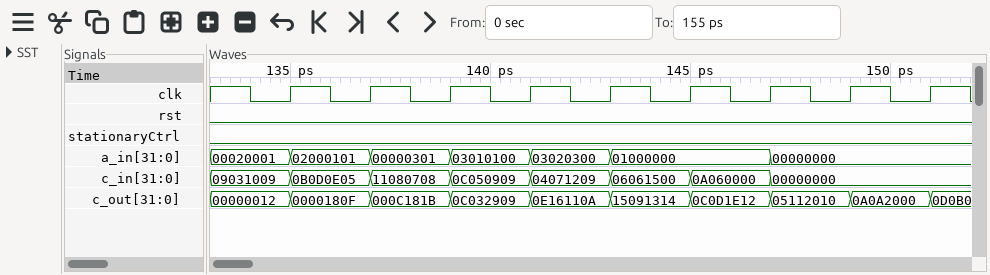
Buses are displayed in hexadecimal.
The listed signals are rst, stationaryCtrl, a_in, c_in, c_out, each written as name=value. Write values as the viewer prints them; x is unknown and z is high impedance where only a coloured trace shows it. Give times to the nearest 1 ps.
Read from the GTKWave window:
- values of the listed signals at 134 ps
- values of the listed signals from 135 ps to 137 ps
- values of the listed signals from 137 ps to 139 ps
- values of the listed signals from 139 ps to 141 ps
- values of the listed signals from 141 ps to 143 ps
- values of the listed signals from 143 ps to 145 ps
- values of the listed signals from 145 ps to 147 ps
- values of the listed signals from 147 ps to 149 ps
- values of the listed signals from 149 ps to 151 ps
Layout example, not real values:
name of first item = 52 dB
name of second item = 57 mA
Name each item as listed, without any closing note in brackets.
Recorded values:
values of the listed signals at 134 ps = rst=0, stationaryCtrl=0, a_in=00020001, c_in=09031009, c_out=00000012
values of the listed signals from 135 ps to 137 ps = rst=0, stationaryCtrl=0, a_in=02000101, c_in=0B0D0E05, c_out=0000180F
values of the listed signals from 137 ps to 139 ps = rst=0, stationaryCtrl=0, a_in=00000301, c_in=11080708, c_out=000C181B
values of the listed signals from 139 ps to 141 ps = rst=0, stationaryCtrl=0, a_in=03010100, c_in=0C050909, c_out=0C032909
values of the listed signals from 141 ps to 143 ps = rst=0, stationaryCtrl=0, a_in=03020300, c_in=04071209, c_out=0E16110A
values of the listed signals from 143 ps to 145 ps = rst=0, stationaryCtrl=0, a_in=01000000, c_in=06061500, c_out=15091314
values of the listed signals from 145 ps to 147 ps = rst=0, stationaryCtrl=0, a_in=01000000, c_in=0A060000, c_out=0C0D1E12
values of the listed signals from 147 ps to 149 ps = rst=0, stationaryCtrl=0, a_in=00000000, c_in=00000000, c_out=05112010
values of the listed signals from 149 ps to 151 ps = rst=0, stationaryCtrl=0, a_in=00000000, c_in=00000000, c_out=0A0A2000
